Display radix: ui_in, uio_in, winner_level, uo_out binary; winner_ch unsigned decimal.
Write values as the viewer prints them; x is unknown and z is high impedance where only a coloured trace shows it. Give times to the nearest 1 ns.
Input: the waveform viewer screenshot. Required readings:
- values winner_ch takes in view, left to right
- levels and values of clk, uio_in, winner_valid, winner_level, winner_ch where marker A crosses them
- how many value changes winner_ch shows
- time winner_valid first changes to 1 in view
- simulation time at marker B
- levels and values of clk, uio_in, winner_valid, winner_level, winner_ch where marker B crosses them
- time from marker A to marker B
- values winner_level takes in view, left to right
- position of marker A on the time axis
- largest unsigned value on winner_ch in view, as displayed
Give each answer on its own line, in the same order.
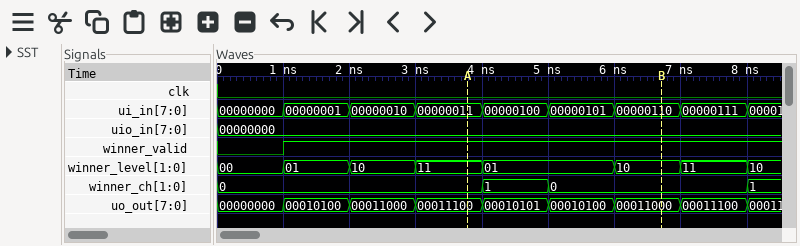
0, 1, 0, 1
clk=0, uio_in=00000000, winner_valid=1, winner_level=11, winner_ch=0
3
1 ns
7 ns
clk=0, uio_in=00000000, winner_valid=1, winner_level=10, winner_ch=0
3 ns
00, 01, 10, 11, 01, 10, 11, 10
4 ns
1
